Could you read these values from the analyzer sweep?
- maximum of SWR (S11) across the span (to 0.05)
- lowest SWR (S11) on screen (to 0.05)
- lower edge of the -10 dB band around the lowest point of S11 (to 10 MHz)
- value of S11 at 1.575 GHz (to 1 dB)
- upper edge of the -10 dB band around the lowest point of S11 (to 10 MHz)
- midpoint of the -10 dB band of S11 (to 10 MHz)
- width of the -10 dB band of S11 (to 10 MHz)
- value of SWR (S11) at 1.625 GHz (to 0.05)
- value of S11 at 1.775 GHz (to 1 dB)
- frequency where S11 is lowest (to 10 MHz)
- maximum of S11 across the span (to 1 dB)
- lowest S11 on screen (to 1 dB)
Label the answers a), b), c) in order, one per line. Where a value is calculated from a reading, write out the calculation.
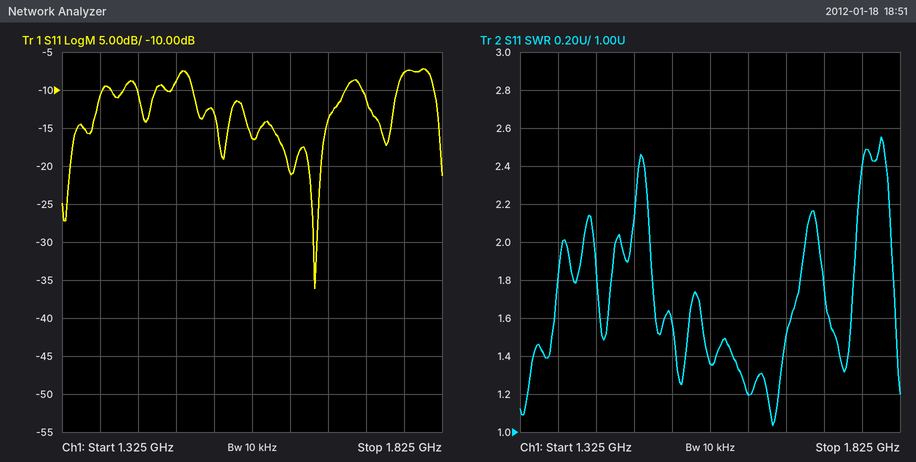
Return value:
a) 2.55
b) 1.05
c) 1.50 GHz
d) -16 dB
e) 1.70 GHz
f) 1.60 GHz
g) 1.70 GHz − 1.50 GHz = 200 MHz
h) 1.20
i) -8 dB
j) 1.66 GHz
k) -7 dB
l) -36 dB
